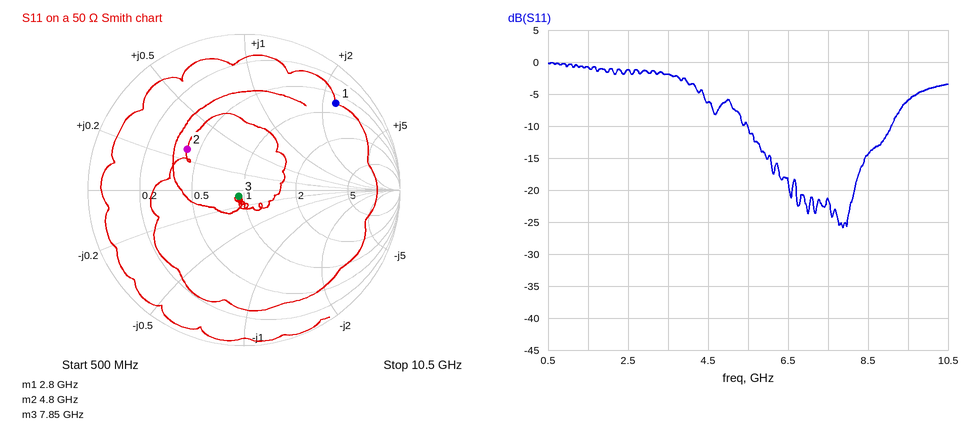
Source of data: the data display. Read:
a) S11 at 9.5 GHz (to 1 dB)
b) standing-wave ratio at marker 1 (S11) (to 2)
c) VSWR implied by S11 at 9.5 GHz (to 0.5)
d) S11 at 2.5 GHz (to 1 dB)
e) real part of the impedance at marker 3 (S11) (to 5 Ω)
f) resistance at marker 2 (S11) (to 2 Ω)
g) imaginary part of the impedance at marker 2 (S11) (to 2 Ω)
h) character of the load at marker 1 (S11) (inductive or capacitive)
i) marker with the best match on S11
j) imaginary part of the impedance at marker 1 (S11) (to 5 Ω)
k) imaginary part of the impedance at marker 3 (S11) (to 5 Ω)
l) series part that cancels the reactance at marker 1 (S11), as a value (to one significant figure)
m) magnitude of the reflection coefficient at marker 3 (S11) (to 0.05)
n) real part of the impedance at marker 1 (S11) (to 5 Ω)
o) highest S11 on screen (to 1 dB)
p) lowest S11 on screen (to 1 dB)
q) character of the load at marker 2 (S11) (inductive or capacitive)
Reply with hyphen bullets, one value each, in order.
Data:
- -6 dB
- 10
- 3.0
- -1 dB
- 45 Ω
- 20 Ω
- +14 Ω
- inductive
- marker 3
- +115 Ω
- -5 Ω
- 500 fF
- 0.05
- 35 Ω
- 0 dB
- -26 dB
- inductive
